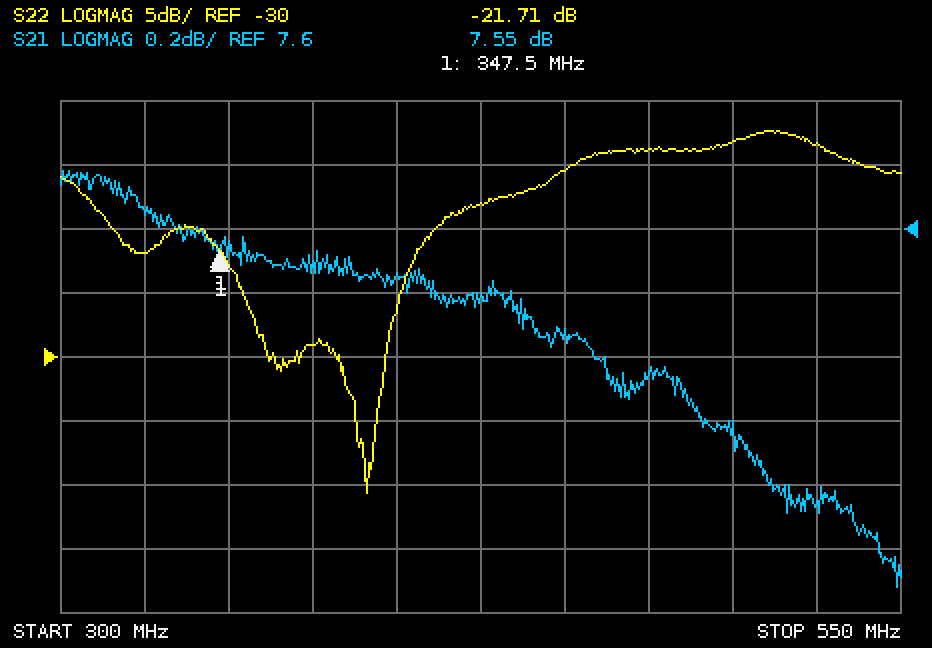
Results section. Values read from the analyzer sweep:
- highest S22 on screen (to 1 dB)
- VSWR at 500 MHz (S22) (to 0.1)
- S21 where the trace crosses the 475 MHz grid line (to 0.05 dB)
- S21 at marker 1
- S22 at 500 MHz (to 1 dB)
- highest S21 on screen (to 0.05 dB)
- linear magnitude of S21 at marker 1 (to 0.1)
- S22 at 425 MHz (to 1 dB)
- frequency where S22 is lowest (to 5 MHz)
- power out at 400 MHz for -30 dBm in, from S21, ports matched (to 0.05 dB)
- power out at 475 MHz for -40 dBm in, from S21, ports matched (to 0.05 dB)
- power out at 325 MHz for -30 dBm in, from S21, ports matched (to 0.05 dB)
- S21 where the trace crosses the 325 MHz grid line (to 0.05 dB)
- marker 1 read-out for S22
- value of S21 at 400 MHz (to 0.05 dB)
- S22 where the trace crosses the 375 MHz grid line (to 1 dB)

-12 dB
1.6
7.15 dB
7.55 dB
-13 dB
7.80 dB
2.4
-18 dB
390 MHz
-22.55 dBm
-32.85 dBm
-22.35 dBm
7.65 dB
-21.71 dB
7.45 dB
-29 dB
